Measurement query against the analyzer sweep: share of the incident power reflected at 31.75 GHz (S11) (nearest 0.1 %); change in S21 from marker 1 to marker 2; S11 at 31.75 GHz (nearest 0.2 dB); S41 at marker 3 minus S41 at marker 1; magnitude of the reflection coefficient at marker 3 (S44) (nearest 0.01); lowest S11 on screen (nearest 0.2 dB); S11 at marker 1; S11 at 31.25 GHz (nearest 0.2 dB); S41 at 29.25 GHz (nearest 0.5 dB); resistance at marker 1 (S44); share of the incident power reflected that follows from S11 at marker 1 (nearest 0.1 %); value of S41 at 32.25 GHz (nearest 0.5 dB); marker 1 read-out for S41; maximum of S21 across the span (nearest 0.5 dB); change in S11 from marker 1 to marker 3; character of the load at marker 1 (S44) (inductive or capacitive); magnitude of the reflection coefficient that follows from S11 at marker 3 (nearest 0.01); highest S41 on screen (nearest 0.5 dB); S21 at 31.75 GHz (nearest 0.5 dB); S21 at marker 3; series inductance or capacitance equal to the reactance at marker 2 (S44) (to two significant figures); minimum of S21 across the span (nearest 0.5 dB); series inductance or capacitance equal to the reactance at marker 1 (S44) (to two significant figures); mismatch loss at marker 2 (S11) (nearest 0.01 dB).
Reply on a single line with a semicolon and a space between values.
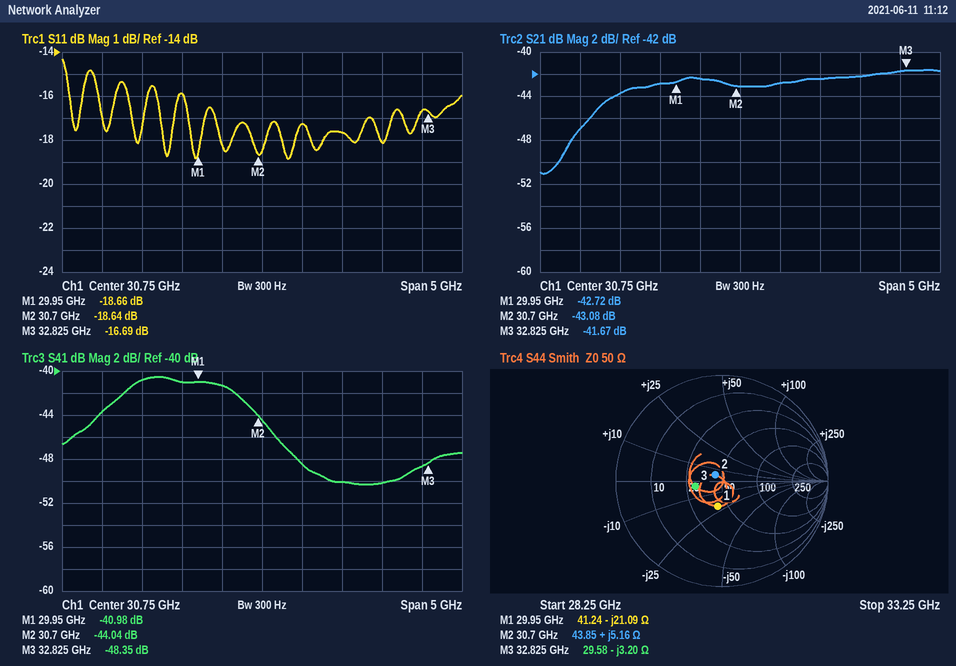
1.7 %; -0.36 dB; -17.6 dB; -7.37 dB; 0.26; -18.8 dB; -18.66 dB; -17.2 dB; -41.0 dB; 41.24 Ω; 1.4 %; -50.0 dB; -40.98 dB; -41.5 dB; 1.97 dB; capacitive; 0.15; -40.5 dB; -42.5 dB; -41.67 dB; 27 pH; -51.0 dB; 250 fF; 0.06 dB
